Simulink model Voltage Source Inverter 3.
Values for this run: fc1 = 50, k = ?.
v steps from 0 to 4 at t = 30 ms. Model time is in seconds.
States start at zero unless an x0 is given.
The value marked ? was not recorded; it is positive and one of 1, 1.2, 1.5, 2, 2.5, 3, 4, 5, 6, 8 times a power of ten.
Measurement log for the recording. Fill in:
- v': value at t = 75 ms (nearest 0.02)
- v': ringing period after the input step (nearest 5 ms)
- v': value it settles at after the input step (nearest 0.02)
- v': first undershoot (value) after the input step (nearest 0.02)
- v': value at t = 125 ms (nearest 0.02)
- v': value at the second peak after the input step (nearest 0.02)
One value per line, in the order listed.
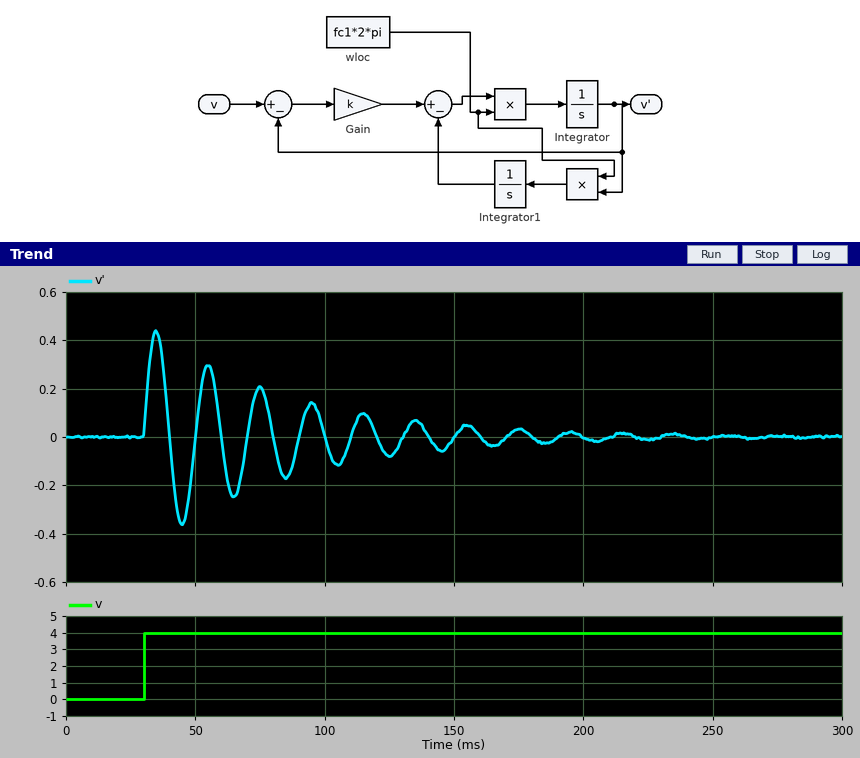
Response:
0.20
20 ms
0.00
-0.36
-0.08
0.30
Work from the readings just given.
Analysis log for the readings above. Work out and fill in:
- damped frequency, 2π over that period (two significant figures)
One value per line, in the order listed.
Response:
0.31 rad/ms
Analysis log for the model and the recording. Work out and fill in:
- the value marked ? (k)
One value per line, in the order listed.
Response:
0.12
